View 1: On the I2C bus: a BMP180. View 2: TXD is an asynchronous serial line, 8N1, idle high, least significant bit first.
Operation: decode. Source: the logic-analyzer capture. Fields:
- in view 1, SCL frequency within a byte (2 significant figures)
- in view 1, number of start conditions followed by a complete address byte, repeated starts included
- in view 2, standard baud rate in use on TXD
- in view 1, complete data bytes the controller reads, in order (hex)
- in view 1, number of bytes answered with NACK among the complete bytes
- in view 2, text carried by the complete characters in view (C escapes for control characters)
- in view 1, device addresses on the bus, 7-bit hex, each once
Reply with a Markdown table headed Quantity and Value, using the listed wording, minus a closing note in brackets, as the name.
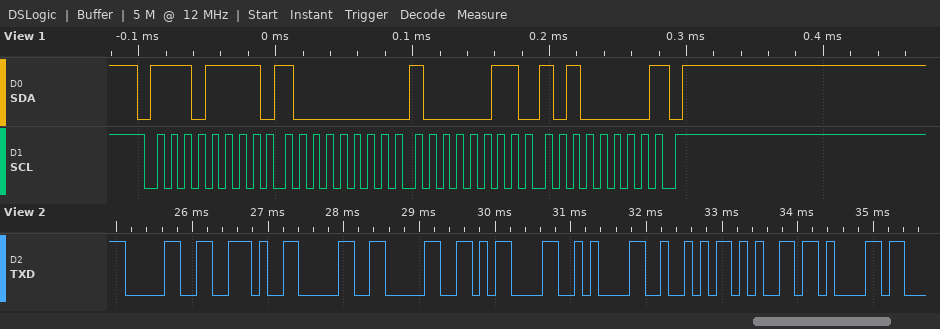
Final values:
| Quantity | Value |
|---|---|
| in view 1, SCL frequency within a byte | 100 kHz |
| in view 1, number of start conditions followed by a complete address byte, repeated starts included | 1 |
| in view 2, standard baud rate in use on TXD | 9600 baud |
| in view 1, complete data bytes the controller reads, in order | 80 83 A0 |
| in view 1, number of bytes answered with NACK among the complete bytes | 1 |
| in view 2, text carried by the complete characters in view | "0.00\r\nRea" |
| in view 1, device addresses on the bus, 7-bit hex, each once | 0x77 |
